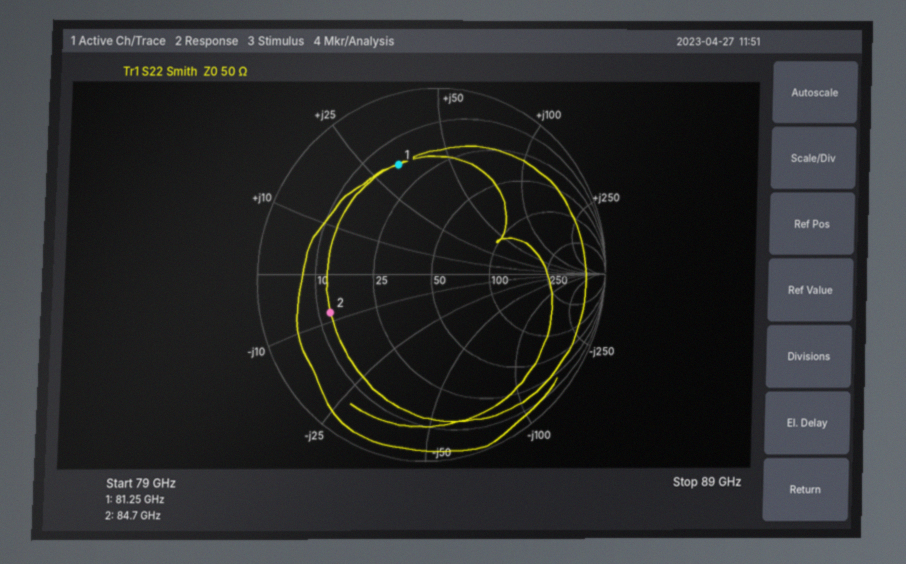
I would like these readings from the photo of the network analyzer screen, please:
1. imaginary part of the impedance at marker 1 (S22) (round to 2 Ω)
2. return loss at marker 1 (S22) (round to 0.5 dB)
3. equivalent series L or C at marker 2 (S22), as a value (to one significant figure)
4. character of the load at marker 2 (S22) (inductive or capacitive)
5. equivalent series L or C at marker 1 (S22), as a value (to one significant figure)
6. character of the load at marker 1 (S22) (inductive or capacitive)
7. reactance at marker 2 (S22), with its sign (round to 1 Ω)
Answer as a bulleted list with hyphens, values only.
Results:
- +32 Ω
- 4.0 dB
- 200 fF
- capacitive
- 60 pH
- inductive
- -8 Ω
